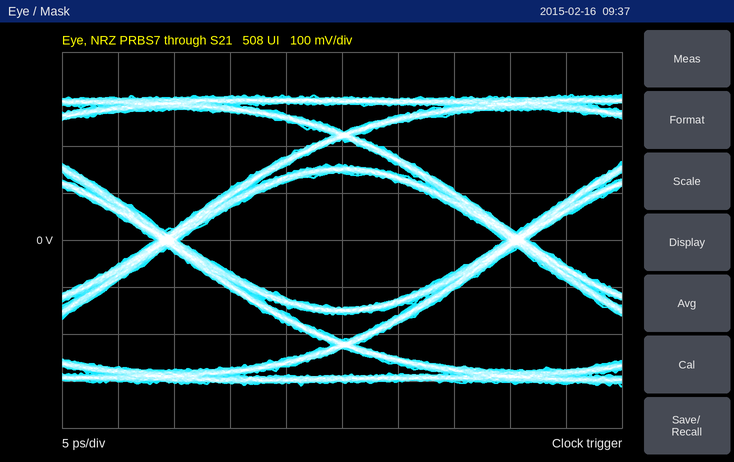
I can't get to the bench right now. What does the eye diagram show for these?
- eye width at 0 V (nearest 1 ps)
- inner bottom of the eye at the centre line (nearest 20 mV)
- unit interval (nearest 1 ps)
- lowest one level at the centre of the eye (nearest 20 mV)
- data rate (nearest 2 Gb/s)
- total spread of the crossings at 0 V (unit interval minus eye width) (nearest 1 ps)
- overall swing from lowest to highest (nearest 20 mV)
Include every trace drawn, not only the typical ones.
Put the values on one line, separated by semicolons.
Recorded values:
29 ps; -140 mV; 31 ps; 140 mV; 32 Gb/s; 2 ps; 620 mV
